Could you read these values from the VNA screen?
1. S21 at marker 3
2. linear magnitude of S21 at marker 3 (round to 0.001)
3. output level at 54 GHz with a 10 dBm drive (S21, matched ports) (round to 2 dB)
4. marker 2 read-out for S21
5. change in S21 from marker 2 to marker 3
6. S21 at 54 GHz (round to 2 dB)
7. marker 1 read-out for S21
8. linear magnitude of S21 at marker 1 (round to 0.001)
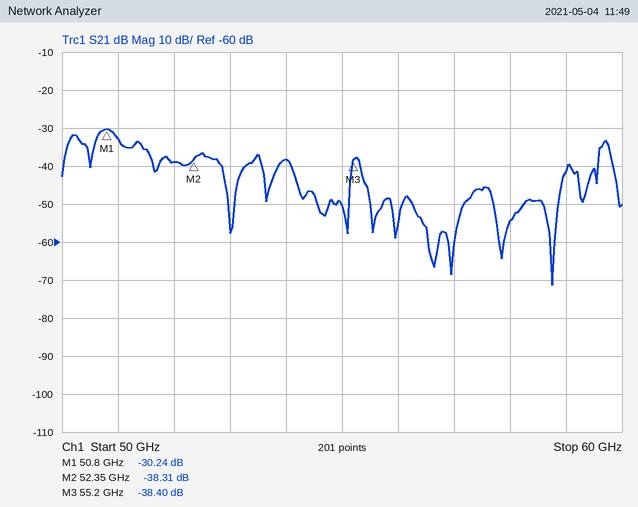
-38.40 dB
0.012
-28 dBm
-38.31 dB
-0.09 dB
-38 dB
-30.24 dB
0.031
